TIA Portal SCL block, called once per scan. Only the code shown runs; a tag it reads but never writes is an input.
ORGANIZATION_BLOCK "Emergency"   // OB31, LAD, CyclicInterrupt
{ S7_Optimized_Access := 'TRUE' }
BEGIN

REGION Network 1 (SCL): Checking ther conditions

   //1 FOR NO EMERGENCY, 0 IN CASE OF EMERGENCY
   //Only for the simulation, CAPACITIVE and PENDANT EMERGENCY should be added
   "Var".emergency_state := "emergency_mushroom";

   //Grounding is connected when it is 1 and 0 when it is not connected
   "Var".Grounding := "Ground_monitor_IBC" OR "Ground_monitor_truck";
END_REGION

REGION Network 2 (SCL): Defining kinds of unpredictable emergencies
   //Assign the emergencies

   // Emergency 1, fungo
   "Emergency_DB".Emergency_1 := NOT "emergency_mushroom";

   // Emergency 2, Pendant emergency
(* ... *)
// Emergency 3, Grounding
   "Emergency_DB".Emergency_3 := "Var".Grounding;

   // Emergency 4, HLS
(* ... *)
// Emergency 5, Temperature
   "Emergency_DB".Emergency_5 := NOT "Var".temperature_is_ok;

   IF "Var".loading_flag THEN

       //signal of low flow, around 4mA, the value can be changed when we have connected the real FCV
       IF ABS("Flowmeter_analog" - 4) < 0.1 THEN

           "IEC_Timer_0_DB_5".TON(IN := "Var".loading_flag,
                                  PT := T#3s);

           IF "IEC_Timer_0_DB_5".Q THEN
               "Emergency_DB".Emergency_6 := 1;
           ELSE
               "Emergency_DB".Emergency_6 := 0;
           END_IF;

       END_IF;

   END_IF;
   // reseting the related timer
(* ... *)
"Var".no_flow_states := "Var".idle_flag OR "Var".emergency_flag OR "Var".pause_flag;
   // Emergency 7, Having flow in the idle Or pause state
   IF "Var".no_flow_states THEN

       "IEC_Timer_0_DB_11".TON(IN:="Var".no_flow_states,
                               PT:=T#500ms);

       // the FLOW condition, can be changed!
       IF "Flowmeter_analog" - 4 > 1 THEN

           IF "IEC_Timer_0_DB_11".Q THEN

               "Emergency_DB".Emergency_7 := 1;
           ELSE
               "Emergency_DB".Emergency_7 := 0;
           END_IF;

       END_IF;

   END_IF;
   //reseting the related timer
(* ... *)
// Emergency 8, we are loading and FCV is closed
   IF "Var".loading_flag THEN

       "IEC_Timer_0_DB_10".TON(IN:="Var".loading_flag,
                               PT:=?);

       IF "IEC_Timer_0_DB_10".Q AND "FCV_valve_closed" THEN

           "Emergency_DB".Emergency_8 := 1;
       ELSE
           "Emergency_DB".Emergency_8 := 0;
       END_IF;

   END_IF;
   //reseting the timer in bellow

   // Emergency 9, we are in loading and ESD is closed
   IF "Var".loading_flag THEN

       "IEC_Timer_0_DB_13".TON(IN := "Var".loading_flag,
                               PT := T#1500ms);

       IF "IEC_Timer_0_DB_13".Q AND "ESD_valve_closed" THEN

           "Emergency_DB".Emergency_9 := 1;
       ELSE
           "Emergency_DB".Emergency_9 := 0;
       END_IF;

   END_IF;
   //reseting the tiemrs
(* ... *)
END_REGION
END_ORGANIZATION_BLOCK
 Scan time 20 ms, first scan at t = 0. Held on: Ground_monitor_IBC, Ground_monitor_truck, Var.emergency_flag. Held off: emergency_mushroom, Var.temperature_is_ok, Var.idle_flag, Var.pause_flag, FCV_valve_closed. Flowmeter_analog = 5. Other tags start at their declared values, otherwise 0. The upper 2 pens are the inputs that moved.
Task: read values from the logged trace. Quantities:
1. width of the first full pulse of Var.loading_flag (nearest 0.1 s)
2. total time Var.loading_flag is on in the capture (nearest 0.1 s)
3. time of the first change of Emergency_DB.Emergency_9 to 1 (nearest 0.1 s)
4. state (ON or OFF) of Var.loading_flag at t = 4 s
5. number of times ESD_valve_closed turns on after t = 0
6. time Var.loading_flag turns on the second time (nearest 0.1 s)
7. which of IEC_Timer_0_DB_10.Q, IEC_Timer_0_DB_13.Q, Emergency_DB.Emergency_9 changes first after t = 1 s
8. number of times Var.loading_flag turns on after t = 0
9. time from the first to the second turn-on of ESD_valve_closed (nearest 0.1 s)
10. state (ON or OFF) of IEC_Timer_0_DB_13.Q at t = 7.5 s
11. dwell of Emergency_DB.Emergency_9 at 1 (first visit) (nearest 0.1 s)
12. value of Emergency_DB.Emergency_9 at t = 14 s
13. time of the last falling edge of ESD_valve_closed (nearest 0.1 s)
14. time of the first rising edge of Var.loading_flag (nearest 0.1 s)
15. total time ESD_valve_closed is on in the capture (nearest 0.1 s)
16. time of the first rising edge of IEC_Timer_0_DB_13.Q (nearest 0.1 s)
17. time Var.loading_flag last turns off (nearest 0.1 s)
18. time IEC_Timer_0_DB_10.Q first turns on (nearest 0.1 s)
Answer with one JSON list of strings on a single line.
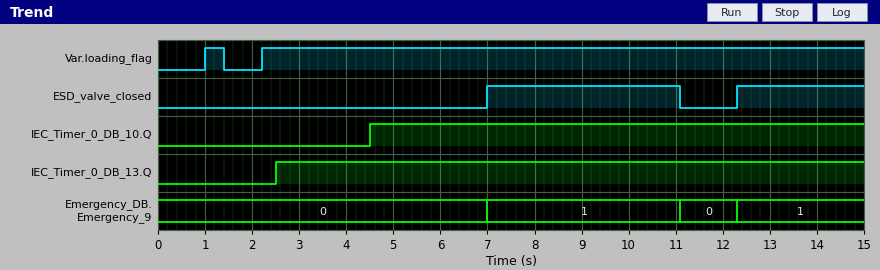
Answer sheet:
["0.4 s", "13.2 s", "7.0 s", "ON", "2", "2.2 s", "IEC_Timer_0_DB_13.Q", "2", "5.3 s", "ON", "4.1 s", "1", "11.1 s", "1.0 s", "6.8 s", "2.5 s", "1.4 s", "4.5 s"]
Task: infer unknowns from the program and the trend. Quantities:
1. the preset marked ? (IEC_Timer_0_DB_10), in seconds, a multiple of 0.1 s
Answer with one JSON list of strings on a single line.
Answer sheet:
["3.5 s"]
